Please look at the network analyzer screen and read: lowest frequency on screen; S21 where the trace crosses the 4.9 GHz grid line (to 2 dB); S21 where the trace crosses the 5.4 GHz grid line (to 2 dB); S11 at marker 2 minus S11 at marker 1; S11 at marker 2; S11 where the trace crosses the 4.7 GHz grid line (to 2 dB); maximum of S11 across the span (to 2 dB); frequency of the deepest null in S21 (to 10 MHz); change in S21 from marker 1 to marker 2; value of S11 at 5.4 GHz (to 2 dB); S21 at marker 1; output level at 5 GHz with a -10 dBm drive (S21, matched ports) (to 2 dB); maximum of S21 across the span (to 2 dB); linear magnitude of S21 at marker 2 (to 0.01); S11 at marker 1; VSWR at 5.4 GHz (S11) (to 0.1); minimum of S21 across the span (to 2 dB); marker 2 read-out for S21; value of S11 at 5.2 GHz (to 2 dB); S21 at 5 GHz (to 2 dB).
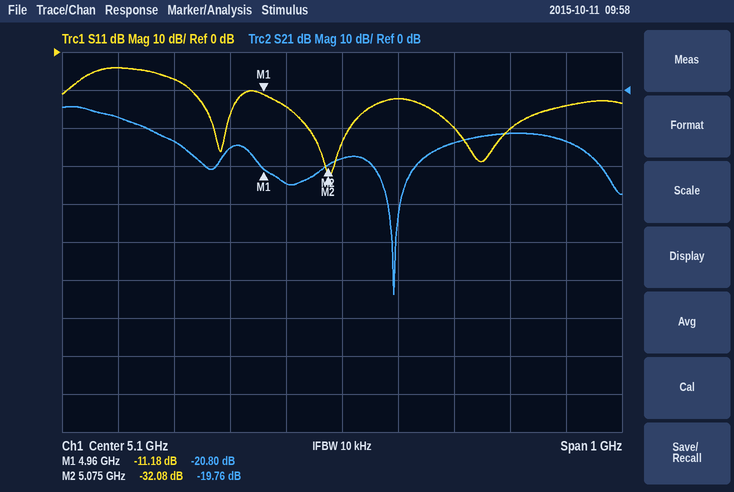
4.6 GHz
-16 dB
-12 dB
-20.90 dB
-32.08 dB
-4 dB
-4 dB
5.19 GHz
1.04 dB
-20 dB
-20.80 dB
-34 dBm
-4 dB
0.10
-11.18 dB
1.2
-54 dB
-19.76 dB
-12 dB
-24 dB
